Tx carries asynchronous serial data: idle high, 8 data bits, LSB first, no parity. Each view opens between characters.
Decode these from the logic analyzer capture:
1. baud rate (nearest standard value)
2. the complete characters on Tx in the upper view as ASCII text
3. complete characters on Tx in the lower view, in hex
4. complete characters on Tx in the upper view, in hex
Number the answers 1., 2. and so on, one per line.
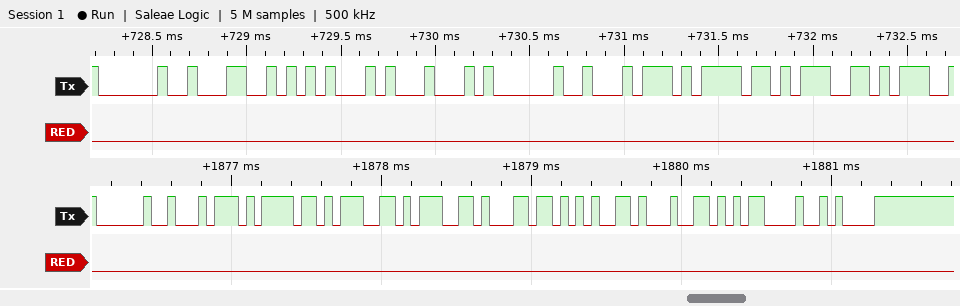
1. 19200 baud
2. " LED tog"
3. 20, 74, 6F, 67, 67, 6C, 65, 64, 0D, 0A
4. 20, 4C, 45, 44, 20, 74, 6F, 67
